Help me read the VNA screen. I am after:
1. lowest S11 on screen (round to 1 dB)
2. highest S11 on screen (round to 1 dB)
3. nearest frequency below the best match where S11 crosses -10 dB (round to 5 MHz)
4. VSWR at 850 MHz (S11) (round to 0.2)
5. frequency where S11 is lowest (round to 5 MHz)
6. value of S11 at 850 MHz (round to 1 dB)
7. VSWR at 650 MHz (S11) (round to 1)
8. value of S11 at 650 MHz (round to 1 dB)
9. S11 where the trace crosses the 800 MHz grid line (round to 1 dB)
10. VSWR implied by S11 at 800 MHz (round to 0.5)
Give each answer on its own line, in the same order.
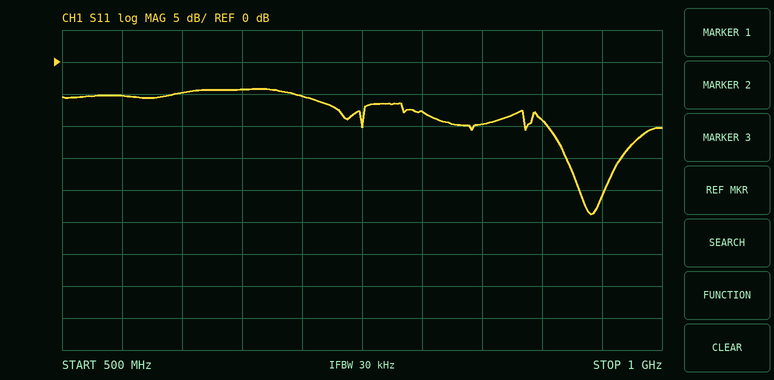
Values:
-24 dB
-4 dB
905 MHz
2.0
940 MHz
-10 dB
4
-4 dB
-8 dB
2.5
